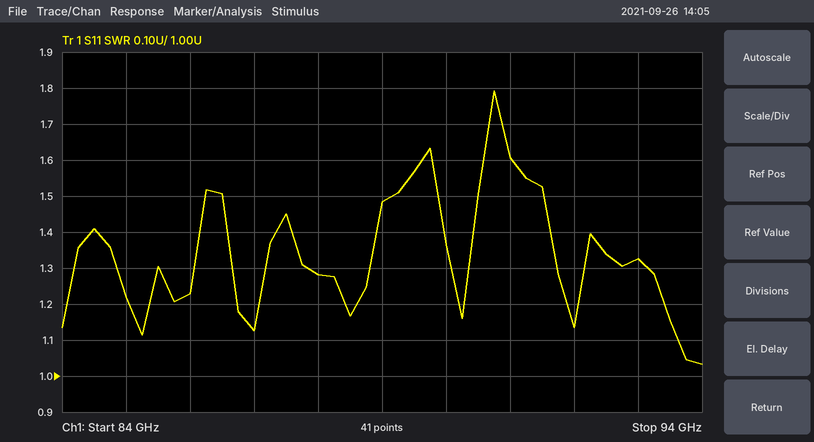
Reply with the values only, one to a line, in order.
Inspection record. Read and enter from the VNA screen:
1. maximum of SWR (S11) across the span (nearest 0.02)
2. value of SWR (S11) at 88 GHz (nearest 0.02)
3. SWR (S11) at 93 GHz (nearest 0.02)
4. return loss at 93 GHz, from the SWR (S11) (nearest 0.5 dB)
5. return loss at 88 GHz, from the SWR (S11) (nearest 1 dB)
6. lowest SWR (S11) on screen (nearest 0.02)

1.80
1.28
1.32
17.0 dB
18 dB
1.04
